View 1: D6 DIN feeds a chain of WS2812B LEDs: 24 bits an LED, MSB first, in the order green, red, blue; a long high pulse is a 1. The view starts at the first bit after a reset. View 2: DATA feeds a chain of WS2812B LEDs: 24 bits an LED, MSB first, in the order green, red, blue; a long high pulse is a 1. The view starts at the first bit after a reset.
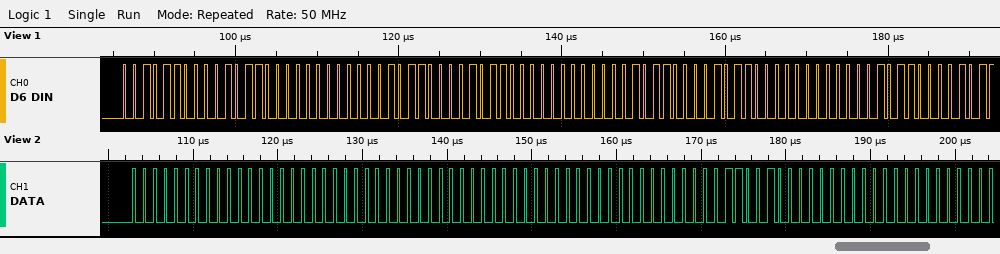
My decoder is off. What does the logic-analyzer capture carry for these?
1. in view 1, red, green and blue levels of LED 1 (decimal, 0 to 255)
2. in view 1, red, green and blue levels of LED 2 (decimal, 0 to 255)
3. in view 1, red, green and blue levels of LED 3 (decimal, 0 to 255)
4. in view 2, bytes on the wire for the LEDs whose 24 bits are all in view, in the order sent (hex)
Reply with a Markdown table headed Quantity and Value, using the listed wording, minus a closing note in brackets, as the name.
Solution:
| Quantity | Value |
|---|---|
| in view 1, red, green and blue levels of LED 1 | 44, 44, 0 |
| in view 1, red, green and blue levels of LED 2 | 44, 44, 0 |
| in view 1, red, green and blue levels of LED 3 | 44, 44, 0 |
| in view 2, bytes on the wire for the LEDs whose 24 bits are all in view, in the order sent | 00 00 00 00 00 00 00 C8 00 |
